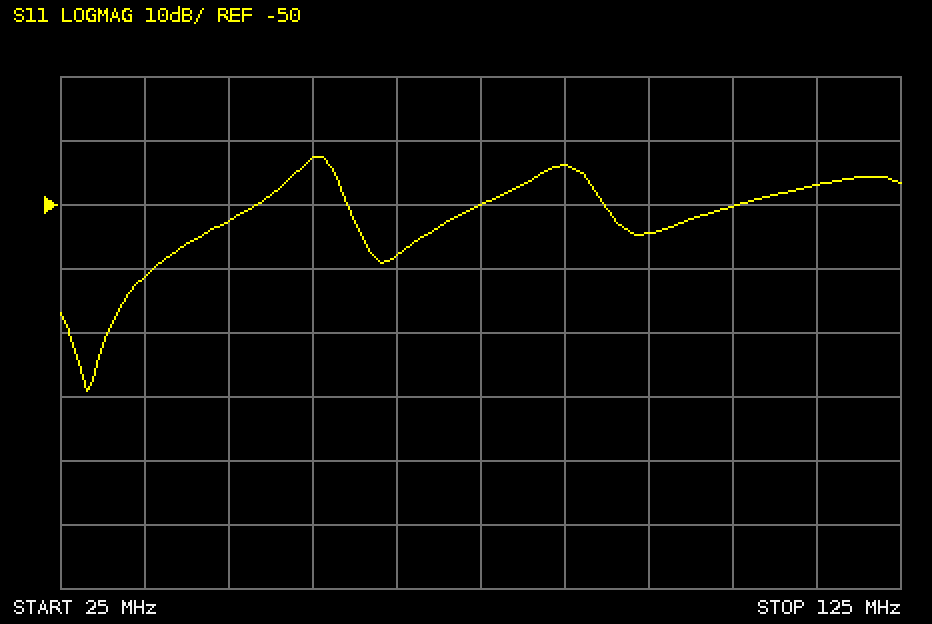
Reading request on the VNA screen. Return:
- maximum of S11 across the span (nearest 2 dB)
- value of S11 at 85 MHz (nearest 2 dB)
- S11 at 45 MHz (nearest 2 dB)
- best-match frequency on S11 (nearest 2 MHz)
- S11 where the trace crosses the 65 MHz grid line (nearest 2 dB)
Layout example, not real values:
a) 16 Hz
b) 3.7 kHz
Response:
a) -42 dB
b) -44 dB
c) -52 dB
d) 28 MHz
e) -58 dB
